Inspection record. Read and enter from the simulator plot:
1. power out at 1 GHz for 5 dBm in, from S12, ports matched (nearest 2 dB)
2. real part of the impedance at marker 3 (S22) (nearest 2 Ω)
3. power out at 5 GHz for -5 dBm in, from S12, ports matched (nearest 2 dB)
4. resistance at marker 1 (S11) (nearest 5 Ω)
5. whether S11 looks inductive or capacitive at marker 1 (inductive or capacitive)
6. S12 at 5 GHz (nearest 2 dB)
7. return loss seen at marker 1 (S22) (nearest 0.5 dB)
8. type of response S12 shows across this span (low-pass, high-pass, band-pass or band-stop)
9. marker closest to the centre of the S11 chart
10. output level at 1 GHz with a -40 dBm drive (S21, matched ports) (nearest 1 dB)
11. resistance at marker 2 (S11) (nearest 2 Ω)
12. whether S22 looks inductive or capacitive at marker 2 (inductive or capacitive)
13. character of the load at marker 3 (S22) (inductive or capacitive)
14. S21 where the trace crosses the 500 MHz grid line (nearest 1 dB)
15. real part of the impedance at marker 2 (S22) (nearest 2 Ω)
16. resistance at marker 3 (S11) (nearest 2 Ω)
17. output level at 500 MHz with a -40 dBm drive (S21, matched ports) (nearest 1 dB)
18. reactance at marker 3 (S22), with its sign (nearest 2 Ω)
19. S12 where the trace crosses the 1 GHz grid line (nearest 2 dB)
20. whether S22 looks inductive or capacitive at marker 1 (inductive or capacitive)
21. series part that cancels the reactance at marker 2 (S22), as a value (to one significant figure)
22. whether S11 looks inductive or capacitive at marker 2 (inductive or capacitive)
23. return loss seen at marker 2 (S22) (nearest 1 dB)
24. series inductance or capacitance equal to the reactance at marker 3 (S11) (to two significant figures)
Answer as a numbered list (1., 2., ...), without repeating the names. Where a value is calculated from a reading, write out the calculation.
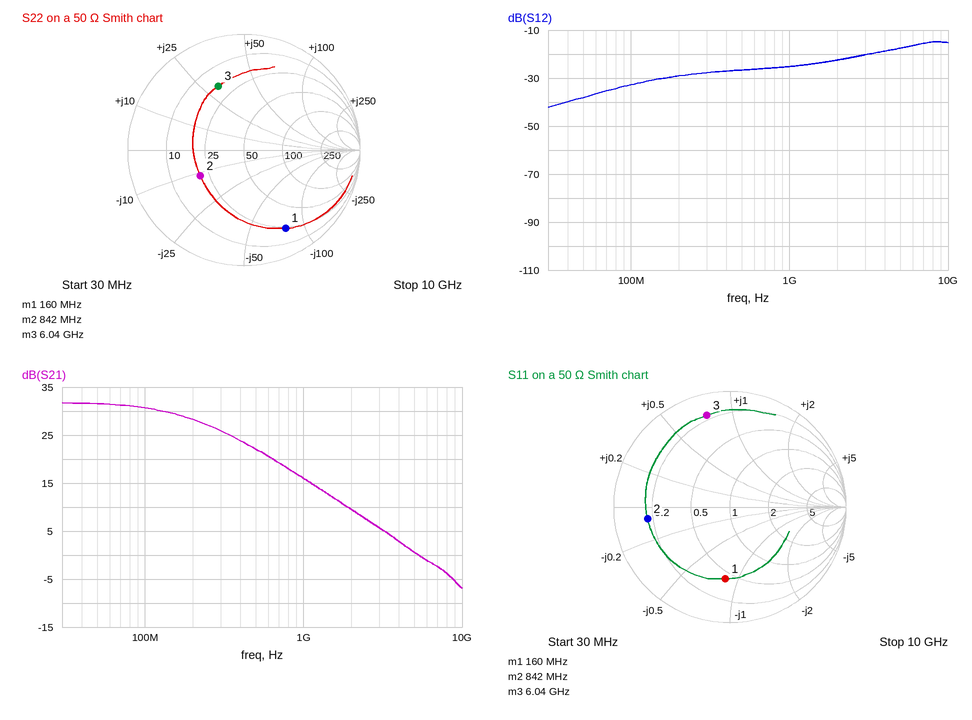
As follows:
1. 5 dBm + (-26 dB) = -20 dBm
2. 18 Ω
3. -5 dBm + (-18 dB) = -22 dBm
4. 20 Ω
5. capacitive
6. -18 dB
7. 2.5 dB
8. high-pass
9. marker 1
10. -40 dBm + (16 dB) = -24 dBm
11. 8 Ω
12. capacitive
13. inductive
14. 22 dB
15. 20 Ω
16. 8 Ω
17. -40 dBm + (22 dB) = -18 dBm
18. +30 Ω
19. -26 dB
20. capacitive
21. L = 12 Ω/(2π × 842 MHz) ≈ 2 nH
22. capacitive
23. 7 dB
24. L = 38 Ω/(2π × 6.04 GHz) ≈ 1.0 nH
